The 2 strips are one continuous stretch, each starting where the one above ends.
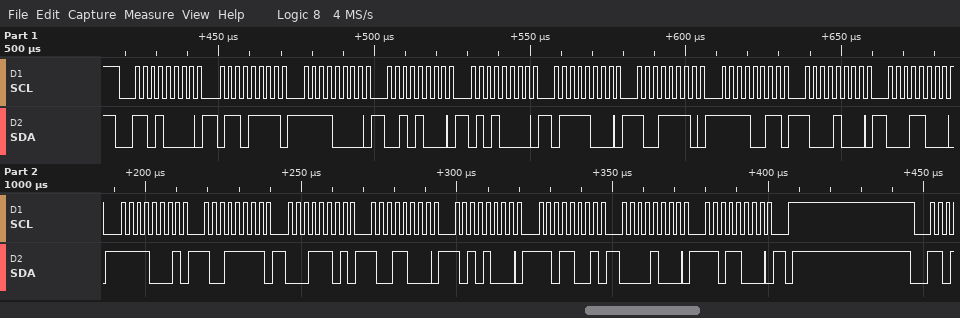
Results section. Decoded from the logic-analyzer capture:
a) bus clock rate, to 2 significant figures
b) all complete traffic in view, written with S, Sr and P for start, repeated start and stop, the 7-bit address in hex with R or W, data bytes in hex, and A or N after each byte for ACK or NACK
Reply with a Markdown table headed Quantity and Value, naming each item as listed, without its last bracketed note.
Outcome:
| Quantity | Value |
|---|---|
| bus clock rate, to 2 significant figures | 400 kHz |
| all complete traffic in view, written with S, Sr and P for start, repeated start and stop, the 7-bit address in hex with R or W, data bytes in hex, and A or N after each byte for ACK or NACK | S 68W A 6F A F0 A 28 A 50 A 78 A 9E A F3 A 88 A 18 A F1 A 9F A 1D A 98 A A8 A D9 A 08 A D8 A P |
